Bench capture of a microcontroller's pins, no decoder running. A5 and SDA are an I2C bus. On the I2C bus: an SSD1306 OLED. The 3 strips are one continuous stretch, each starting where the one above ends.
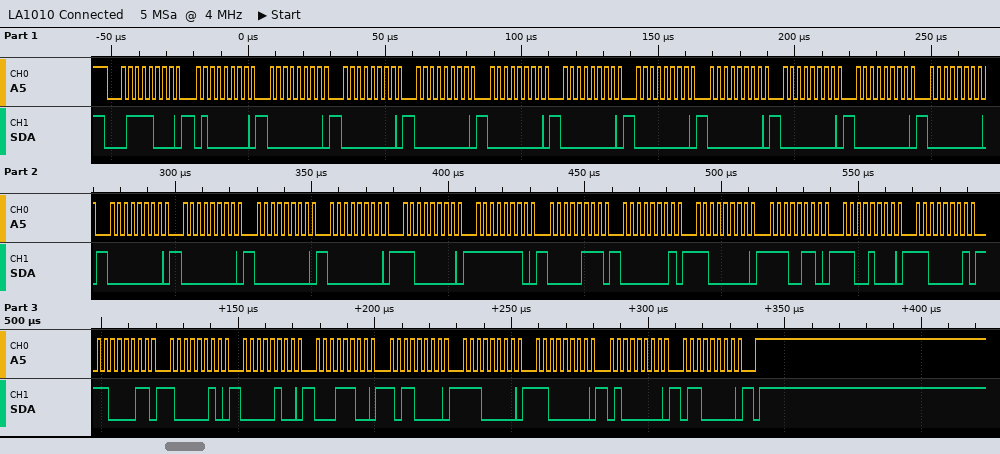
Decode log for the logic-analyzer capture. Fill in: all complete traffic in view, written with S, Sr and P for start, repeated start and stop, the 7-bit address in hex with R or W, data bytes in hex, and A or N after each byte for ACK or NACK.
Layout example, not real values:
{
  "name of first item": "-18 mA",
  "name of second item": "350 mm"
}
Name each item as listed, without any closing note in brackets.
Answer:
{
  "all complete traffic in view, written with S, Sr and P for start, repeated start and stop, the 7-bit address in hex with R or W, data bytes in hex, and A or N after each byte for ACK or NACK": "S 3CW A 40 A 00 A 00 A 00 A 00 A 00 A 00 A 00 A 00 A 00 A 00 A 00 A 00 A 00 A 00 A C0 A FE A 07 A 01 A C0 A E6 A C8 A C1 A C3 A 82 A 04 A 1C A B0 A E0 A C0 A 40 A 60 A P"
}
